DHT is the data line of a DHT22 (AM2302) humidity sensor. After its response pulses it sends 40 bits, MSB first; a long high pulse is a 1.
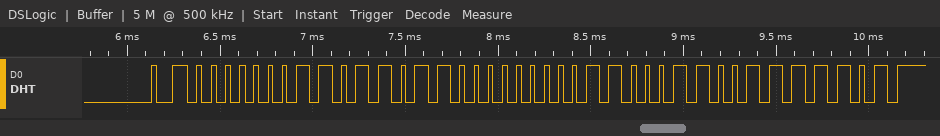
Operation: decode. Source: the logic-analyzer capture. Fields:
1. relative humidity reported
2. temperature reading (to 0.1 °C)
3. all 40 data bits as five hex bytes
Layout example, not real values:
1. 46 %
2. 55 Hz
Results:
1. 43.8 %
2. 19.8 °C
3. 01 B6 00 C6 7D
